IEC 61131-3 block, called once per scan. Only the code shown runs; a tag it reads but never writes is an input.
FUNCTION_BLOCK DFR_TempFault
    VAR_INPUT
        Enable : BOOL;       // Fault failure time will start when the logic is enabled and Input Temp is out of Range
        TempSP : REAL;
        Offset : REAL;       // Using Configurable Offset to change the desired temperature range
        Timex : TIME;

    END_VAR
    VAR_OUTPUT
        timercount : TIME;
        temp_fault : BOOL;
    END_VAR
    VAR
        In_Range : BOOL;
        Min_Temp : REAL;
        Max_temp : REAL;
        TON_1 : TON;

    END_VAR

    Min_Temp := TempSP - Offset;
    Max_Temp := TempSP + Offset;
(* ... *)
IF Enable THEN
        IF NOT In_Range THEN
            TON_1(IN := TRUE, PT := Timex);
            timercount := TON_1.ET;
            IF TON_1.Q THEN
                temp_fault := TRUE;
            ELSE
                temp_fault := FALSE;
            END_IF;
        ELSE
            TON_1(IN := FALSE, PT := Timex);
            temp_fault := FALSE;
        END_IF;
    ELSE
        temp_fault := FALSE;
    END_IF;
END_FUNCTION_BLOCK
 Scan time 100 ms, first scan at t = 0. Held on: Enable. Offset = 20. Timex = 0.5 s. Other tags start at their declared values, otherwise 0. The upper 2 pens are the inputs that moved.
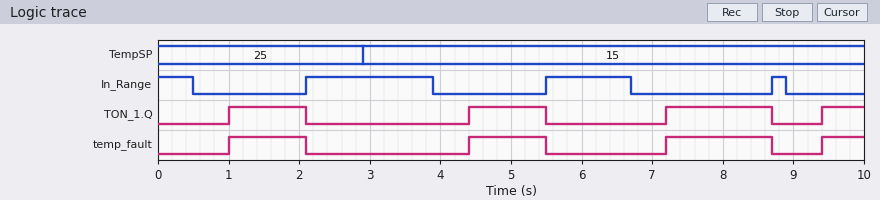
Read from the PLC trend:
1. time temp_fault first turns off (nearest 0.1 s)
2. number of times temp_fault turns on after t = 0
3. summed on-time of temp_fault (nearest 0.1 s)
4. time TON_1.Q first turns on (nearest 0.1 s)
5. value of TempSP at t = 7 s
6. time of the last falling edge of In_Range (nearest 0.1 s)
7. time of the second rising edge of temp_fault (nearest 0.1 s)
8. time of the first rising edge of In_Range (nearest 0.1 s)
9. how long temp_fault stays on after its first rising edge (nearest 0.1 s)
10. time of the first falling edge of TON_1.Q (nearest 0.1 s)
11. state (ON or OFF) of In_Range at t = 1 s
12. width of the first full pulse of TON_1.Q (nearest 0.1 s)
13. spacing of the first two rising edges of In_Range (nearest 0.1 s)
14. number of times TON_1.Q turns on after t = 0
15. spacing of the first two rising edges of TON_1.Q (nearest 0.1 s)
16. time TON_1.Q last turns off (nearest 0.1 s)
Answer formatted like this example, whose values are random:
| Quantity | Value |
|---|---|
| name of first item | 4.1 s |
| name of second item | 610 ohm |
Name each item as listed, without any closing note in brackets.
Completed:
| Quantity | Value |
|---|---|
| time temp_fault first turns off | 2.1 s |
| number of times temp_fault turns on after t = 0 | 4 |
| summed on-time of temp_fault | 4.3 s |
| time TON_1.Q first turns on | 1.0 s |
| value of TempSP at t = 7 s | 15 |
| time of the last falling edge of In_Range | 8.9 s |
| time of the second rising edge of temp_fault | 4.4 s |
| time of the first rising edge of In_Range | 2.1 s |
| how long temp_fault stays on after its first rising edge | 1.1 s |
| time of the first falling edge of TON_1.Q | 2.1 s |
| state (ON or OFF) of In_Range at t = 1 s | OFF |
| width of the first full pulse of TON_1.Q | 1.1 s |
| spacing of the first two rising edges of In_Range | 3.4 s |
| number of times TON_1.Q turns on after t = 0 | 4 |
| spacing of the first two rising edges of TON_1.Q | 3.4 s |
| time TON_1.Q last turns off | 8.7 s |
